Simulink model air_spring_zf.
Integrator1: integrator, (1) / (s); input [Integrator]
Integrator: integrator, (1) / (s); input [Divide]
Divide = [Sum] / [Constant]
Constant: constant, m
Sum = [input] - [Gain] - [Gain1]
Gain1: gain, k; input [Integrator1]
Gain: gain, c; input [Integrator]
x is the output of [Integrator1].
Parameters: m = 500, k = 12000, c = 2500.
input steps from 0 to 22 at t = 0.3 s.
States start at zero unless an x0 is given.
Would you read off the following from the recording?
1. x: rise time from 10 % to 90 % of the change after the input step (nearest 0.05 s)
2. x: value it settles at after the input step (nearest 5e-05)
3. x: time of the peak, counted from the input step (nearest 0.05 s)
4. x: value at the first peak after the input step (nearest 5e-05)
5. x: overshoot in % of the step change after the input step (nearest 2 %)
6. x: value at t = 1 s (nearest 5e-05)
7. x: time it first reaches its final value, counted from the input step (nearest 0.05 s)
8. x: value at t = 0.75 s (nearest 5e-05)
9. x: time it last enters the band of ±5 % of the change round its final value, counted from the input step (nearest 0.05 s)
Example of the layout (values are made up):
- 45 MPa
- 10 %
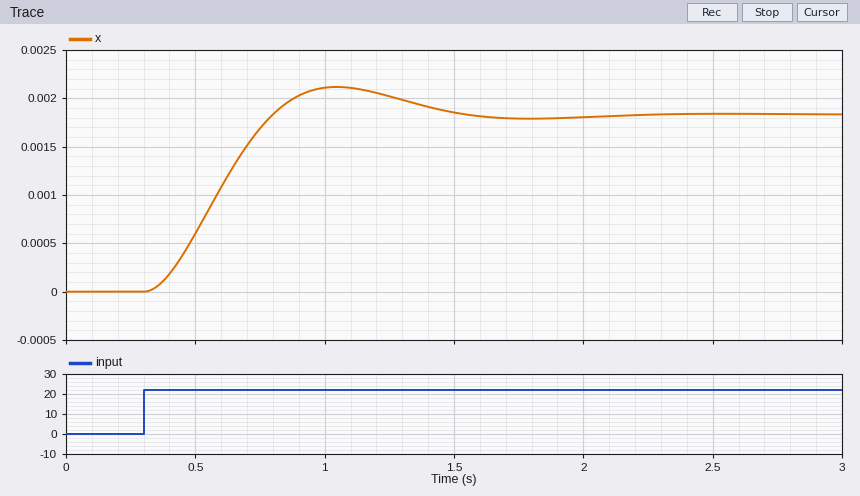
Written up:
- 0.35 s
- 0.00185
- 0.75 s
- 0.00210
- 16 %
- 0.00210
- 0.50 s
- 0.00170
- 1.10 s
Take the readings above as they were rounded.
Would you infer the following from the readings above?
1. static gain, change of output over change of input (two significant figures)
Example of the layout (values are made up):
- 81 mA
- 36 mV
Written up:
- 0.000084
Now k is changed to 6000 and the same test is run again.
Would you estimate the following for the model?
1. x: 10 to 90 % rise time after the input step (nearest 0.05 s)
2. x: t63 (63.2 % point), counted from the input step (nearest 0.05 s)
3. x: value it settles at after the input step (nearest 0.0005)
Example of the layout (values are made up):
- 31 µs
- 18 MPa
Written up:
- 0.65 s
- 0.50 s
- 0.0035
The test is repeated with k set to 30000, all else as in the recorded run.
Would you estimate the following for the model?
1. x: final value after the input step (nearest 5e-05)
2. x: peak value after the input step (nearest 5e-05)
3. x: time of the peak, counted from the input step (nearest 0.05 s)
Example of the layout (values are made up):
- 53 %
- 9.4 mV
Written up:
- 0.00075
- 0.00100
- 0.45 s
